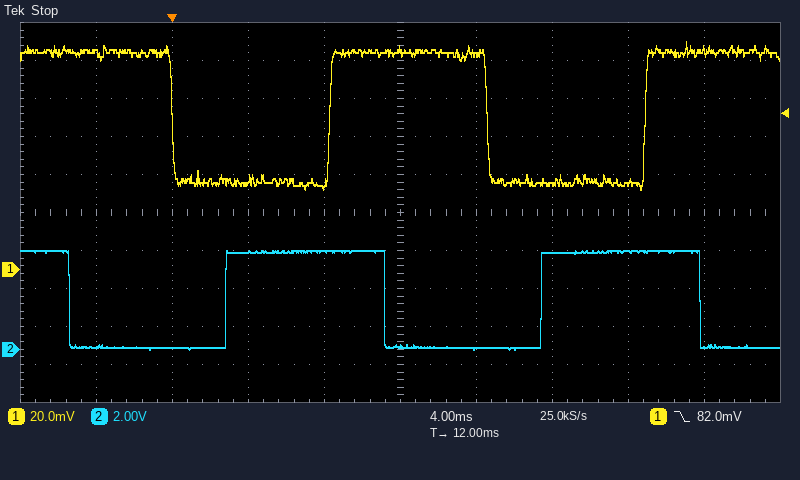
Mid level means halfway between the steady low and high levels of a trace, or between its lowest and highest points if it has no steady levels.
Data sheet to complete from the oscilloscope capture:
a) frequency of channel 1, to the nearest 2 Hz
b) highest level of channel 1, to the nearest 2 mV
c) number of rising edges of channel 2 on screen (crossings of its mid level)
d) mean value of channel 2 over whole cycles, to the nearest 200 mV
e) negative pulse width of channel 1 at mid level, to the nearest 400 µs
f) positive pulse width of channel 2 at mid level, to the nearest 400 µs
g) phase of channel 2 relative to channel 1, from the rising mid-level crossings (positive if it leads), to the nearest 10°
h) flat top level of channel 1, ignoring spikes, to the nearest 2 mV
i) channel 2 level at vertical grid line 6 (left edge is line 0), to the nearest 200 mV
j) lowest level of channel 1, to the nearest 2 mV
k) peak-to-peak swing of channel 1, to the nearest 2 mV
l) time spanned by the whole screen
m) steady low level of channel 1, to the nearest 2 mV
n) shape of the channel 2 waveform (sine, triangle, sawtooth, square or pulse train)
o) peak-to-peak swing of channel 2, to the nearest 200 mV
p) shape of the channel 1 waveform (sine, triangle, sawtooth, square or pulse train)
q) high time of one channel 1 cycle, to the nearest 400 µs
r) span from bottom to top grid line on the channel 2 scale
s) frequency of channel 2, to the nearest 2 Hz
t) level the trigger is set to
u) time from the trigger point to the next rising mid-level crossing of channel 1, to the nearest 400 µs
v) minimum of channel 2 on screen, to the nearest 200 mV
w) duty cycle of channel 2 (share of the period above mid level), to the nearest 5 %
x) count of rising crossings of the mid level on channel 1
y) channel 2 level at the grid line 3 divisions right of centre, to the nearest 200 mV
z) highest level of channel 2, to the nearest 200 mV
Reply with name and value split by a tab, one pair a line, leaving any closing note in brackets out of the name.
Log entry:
frequency of channel 1, to the nearest 2 Hz	60 Hz
highest level of channel 1, to the nearest 2 mV	120 mV
number of rising edges of channel 2 on screen	2
mean value of channel 2 over whole cycles, to the nearest 200 mV	2.6 V
negative pulse width of channel 1 at mid level, to the nearest 400 µs	8.4 ms
positive pulse width of channel 2 at mid level, to the nearest 400 µs	8.4 ms
phase of channel 2 relative to channel 1, from the rising mid-level crossings (positive if it leads), to the nearest 10°	+120°
flat top level of channel 1, ignoring spikes, to the nearest 2 mV	114 mV
channel 2 level at vertical grid line 6 (left edge is line 0), to the nearest 200 mV	0.0 V
lowest level of channel 1, to the nearest 2 mV	42 mV
peak-to-peak swing of channel 1, to the nearest 2 mV	78 mV
time spanned by the whole screen	40 ms
steady low level of channel 1, to the nearest 2 mV	46 mV
shape of the channel 2 waveform	square
peak-to-peak swing of channel 2, to the nearest 200 mV	5.2 V
shape of the channel 1 waveform	square
high time of one channel 1 cycle, to the nearest 400 µs	8.4 ms
span from bottom to top grid line on the channel 2 scale	20 V
frequency of channel 2, to the nearest 2 Hz	60 Hz
level the trigger is set to	82.0 mV
time from the trigger point to the next rising mid-level crossing of channel 1, to the nearest 400 µs	8.4 ms
minimum of channel 2 on screen, to the nearest 200 mV	0.0 V
duty cycle of channel 2 (share of the period above mid level), to the nearest 5 %	50 %
count of rising crossings of the mid level on channel 1	2
channel 2 level at the grid line 3 divisions right of centre, to the nearest 200 mV	5.2 V
highest level of channel 2, to the nearest 200 mV	5.2 V
